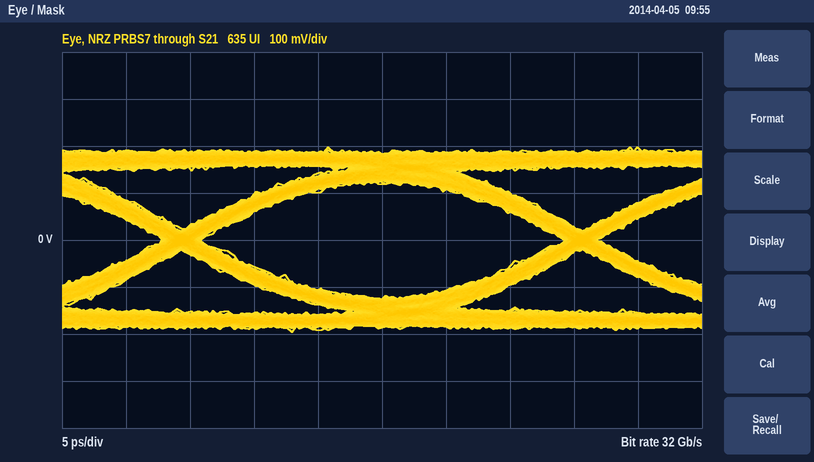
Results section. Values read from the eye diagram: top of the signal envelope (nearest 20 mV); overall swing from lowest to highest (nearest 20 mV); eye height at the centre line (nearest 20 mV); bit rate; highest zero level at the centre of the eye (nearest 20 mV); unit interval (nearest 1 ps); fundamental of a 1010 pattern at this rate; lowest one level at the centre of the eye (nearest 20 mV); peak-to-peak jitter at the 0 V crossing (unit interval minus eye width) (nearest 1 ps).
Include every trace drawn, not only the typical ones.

200 mV
400 mV
240 mV
32 Gb/s
-120 mV
31 ps
16 GHz
120 mV
3 ps
